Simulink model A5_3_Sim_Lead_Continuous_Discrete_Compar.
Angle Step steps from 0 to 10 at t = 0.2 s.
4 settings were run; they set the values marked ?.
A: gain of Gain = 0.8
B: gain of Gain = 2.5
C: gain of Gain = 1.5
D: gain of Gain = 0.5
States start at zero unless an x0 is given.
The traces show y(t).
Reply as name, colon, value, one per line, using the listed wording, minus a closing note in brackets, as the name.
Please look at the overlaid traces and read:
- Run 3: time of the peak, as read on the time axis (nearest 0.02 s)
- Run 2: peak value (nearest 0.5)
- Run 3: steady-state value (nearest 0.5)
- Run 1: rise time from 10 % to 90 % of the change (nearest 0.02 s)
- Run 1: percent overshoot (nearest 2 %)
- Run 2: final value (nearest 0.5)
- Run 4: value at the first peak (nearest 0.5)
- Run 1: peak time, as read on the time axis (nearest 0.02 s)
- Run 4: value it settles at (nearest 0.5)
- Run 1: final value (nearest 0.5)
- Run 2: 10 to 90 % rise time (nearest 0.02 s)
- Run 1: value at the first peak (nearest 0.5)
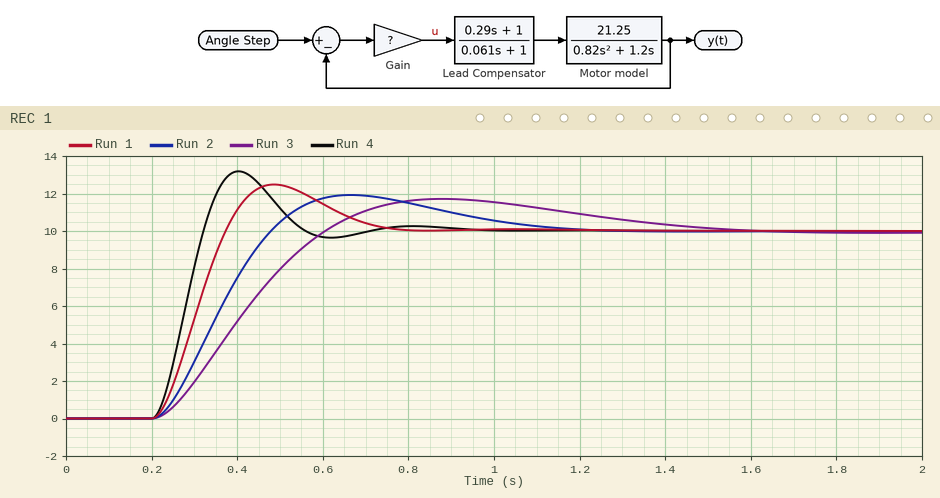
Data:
Run 3: time of the peak, as read on the time axis: 0.88 s
Run 2: peak value: 12.0
Run 3: steady-state value: 10.0
Run 1: rise time from 10 % to 90 % of the change: 0.12 s
Run 1: percent overshoot: 24 %
Run 2: final value: 10.0
Run 4: value at the first peak: 13.0
Run 1: peak time, as read on the time axis: 0.48 s
Run 4: value it settles at: 10.0
Run 1: final value: 10.0
Run 2: 10 to 90 % rise time: 0.20 s
Run 1: value at the first peak: 12.5
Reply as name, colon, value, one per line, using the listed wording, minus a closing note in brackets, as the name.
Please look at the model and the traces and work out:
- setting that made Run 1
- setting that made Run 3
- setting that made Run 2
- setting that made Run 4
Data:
setting that made Run 1: C
setting that made Run 3: D
setting that made Run 2: A
setting that made Run 4: B
